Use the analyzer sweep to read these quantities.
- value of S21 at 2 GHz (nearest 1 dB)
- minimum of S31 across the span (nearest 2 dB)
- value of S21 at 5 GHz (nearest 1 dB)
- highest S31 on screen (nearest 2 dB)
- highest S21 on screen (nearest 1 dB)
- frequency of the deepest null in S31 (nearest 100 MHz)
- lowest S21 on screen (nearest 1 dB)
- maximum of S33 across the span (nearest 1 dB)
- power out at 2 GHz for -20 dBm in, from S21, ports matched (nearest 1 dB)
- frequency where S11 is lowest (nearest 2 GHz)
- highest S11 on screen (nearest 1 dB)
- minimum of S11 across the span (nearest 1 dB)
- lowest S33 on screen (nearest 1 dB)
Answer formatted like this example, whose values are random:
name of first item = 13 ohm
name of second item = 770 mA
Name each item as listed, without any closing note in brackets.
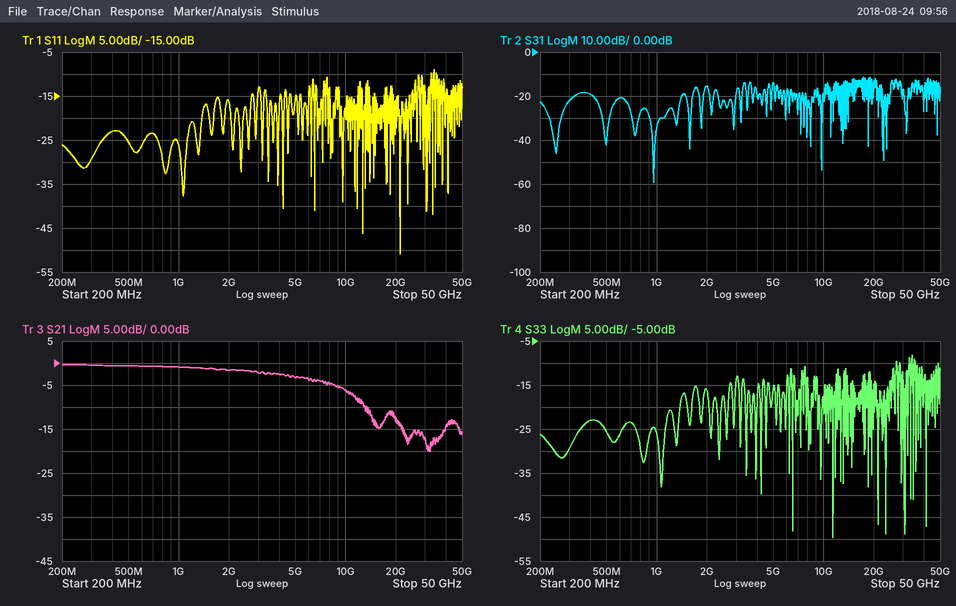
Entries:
value of S21 at 2 GHz = -2 dB
minimum of S31 across the span = -60 dB
value of S21 at 5 GHz = -3 dB
highest S31 on screen = -12 dB
highest S21 on screen = 0 dB
frequency of the deepest null in S31 = 1.0 GHz
lowest S21 on screen = -20 dB
maximum of S33 across the span = -8 dB
power out at 2 GHz for -20 dBm in, from S21, ports matched = -22 dBm
frequency where S11 is lowest = 22 GHz
highest S11 on screen = -9 dB
minimum of S11 across the span = -51 dB
lowest S33 on screen = -50 dB
